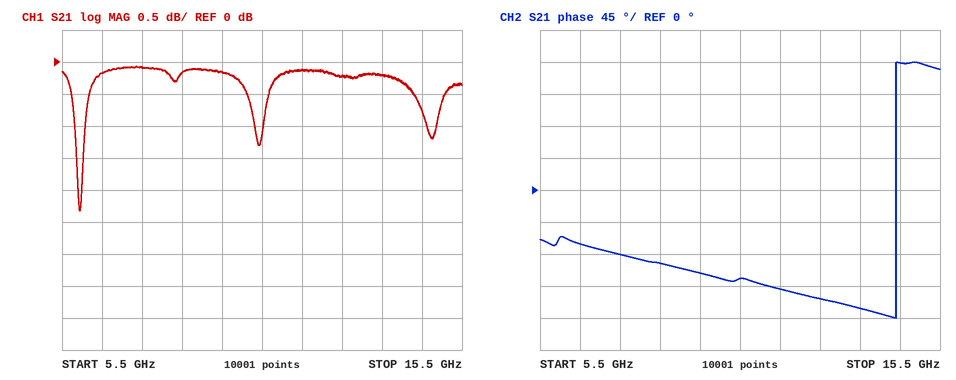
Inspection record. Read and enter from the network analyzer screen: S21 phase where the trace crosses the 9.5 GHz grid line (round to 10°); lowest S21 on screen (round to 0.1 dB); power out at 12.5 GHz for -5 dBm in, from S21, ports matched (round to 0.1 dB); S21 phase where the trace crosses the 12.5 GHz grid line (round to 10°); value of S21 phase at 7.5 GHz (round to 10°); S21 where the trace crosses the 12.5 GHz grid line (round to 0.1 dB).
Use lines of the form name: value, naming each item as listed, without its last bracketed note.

S21 phase where the trace crosses the 9.5 GHz grid line: -120°
lowest S21 on screen: -2.3 dB
power out at 12.5 GHz for -5 dBm in, from S21, ports matched: -5.2 dBm
S21 phase where the trace crosses the 12.5 GHz grid line: -150°
value of S21 phase at 7.5 GHz: -90°
S21 where the trace crosses the 12.5 GHz grid line: -0.2 dB
